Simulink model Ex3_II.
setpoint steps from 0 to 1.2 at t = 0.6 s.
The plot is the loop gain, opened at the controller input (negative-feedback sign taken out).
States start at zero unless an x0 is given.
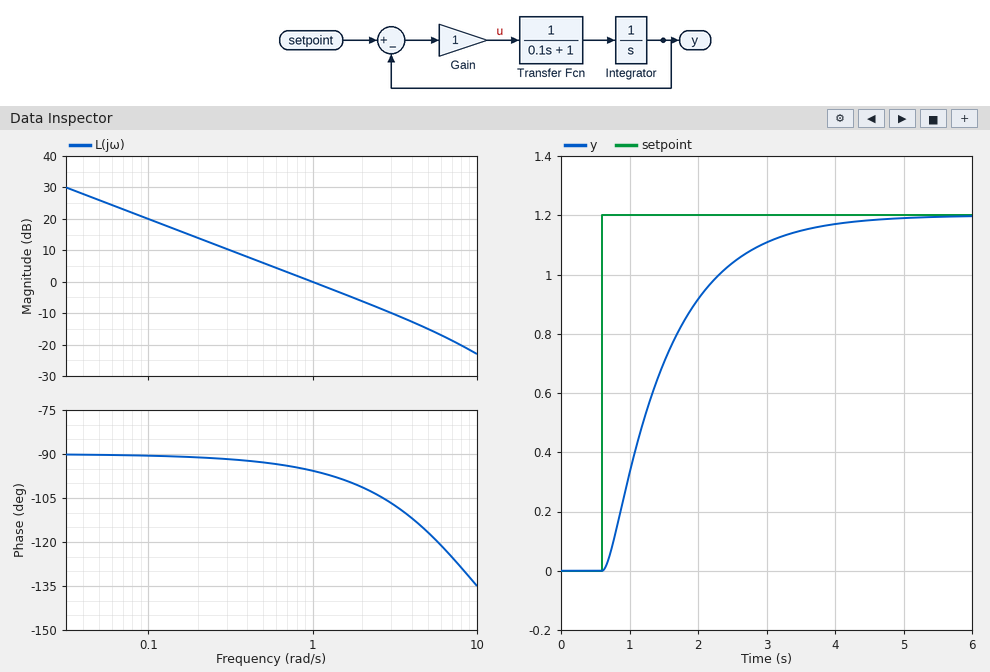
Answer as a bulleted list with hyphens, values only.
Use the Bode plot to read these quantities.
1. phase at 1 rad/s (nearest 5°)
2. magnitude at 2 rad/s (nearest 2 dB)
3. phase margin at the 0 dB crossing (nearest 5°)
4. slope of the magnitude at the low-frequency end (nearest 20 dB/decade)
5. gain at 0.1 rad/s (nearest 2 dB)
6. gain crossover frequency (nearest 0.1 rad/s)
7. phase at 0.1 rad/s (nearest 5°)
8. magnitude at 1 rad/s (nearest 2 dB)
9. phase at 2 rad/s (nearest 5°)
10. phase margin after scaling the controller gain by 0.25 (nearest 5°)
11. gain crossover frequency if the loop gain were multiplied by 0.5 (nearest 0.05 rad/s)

- -95°
- -6 dB
- 85°
- -20 dB/decade
- 20 dB
- 1.0 rad/s
- -90°
- 0 dB
- -100°
- 90°
- 0.50 rad/s
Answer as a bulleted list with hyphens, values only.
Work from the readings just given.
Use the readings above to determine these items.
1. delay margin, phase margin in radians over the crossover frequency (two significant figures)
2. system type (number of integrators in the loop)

- 1.5 s
- 1
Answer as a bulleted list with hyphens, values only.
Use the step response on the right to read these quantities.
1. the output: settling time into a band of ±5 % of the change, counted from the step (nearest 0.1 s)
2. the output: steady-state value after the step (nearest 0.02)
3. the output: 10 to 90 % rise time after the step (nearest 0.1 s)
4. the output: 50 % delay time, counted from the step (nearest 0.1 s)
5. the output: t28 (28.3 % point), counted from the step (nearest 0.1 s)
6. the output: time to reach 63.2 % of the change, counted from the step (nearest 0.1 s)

- 2.8 s
- 1.20
- 2.0 s
- 0.7 s
- 0.4 s
- 1.0 s
